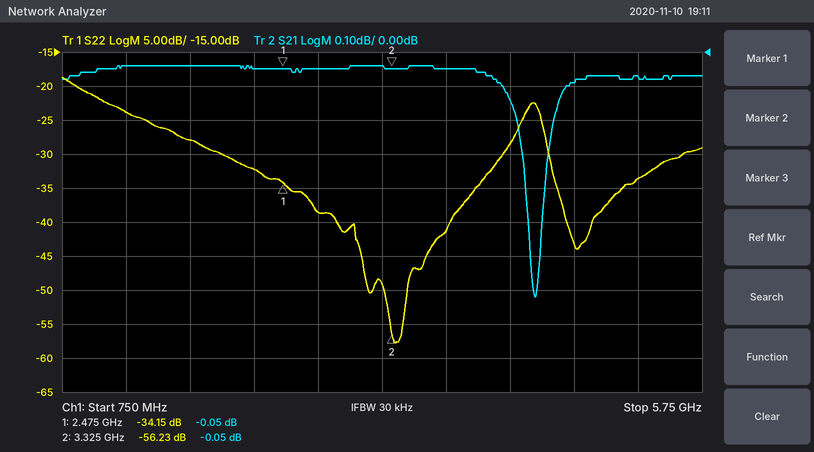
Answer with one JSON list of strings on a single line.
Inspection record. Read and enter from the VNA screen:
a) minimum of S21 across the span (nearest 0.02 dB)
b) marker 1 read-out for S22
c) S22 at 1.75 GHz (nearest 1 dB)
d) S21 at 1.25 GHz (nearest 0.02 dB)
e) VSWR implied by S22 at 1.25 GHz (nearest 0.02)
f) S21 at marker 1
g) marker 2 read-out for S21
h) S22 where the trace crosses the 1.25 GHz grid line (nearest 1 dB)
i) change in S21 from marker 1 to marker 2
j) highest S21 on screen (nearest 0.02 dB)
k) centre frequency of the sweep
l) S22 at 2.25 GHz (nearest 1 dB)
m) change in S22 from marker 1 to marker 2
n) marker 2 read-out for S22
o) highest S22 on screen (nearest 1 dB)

["-0.72 dB", "-34.15 dB", "-28 dB", "-0.04 dB", "1.14", "-0.05 dB", "-0.05 dB", "-24 dB", "0.00 dB", "-0.04 dB", "3.25 GHz", "-32 dB", "-22.08 dB", "-56.23 dB", "-19 dB"]
